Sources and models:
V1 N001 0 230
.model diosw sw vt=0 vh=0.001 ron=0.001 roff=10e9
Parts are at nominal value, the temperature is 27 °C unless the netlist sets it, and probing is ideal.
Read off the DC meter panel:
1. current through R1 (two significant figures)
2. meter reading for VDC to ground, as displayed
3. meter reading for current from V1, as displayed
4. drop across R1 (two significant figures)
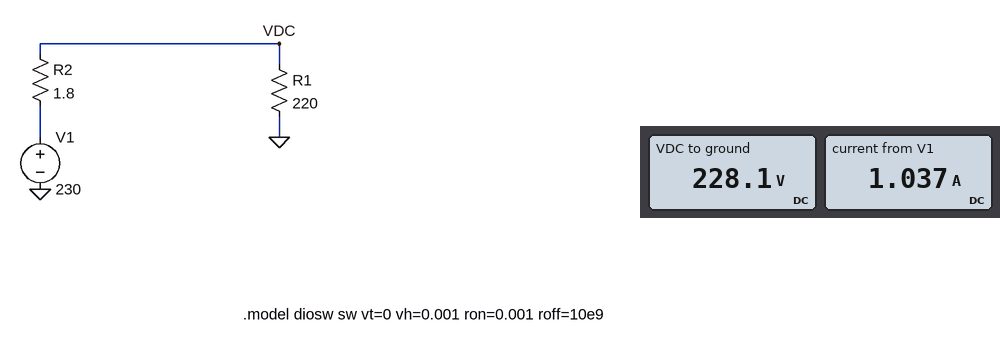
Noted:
1.0 A
228.1 V
1.037 A
230 V
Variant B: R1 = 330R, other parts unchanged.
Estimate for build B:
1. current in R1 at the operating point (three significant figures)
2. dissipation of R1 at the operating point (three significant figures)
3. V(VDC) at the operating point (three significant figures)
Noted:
693 mA
159 W
229 V
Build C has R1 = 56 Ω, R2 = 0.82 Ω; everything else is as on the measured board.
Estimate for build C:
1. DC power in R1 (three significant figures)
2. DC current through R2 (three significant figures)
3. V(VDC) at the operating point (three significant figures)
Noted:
918 W
4.05 A
227 V
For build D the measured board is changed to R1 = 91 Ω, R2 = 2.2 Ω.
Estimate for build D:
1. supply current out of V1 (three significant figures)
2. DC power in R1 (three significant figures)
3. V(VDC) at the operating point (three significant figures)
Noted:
2.47 A
554 W
225 V
